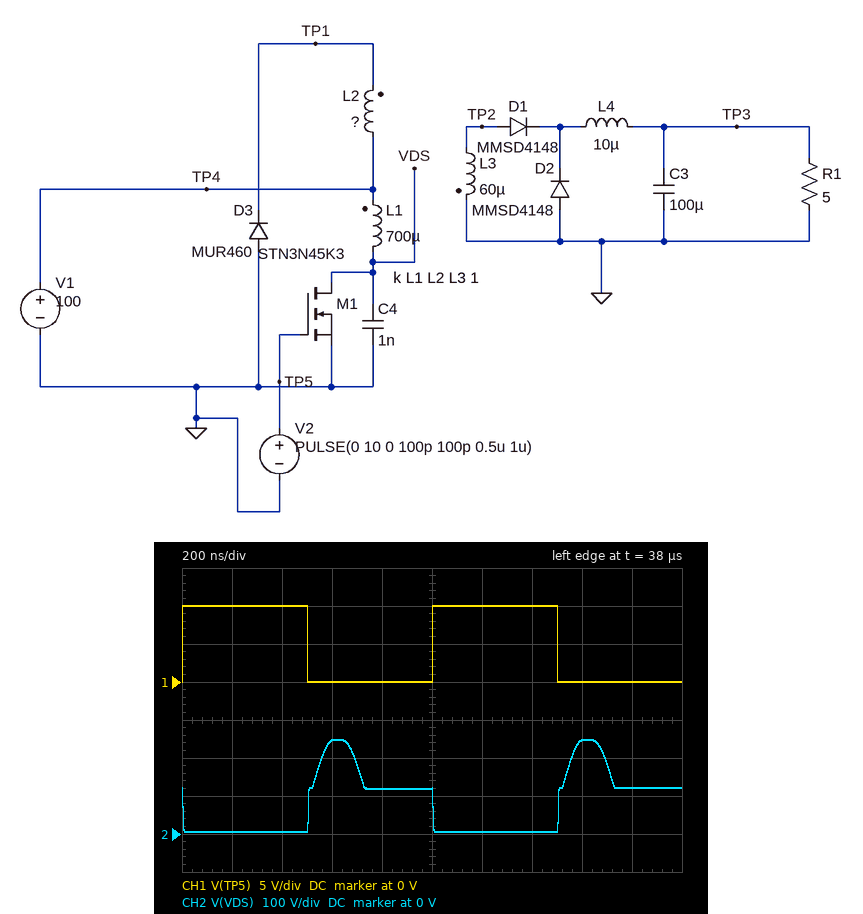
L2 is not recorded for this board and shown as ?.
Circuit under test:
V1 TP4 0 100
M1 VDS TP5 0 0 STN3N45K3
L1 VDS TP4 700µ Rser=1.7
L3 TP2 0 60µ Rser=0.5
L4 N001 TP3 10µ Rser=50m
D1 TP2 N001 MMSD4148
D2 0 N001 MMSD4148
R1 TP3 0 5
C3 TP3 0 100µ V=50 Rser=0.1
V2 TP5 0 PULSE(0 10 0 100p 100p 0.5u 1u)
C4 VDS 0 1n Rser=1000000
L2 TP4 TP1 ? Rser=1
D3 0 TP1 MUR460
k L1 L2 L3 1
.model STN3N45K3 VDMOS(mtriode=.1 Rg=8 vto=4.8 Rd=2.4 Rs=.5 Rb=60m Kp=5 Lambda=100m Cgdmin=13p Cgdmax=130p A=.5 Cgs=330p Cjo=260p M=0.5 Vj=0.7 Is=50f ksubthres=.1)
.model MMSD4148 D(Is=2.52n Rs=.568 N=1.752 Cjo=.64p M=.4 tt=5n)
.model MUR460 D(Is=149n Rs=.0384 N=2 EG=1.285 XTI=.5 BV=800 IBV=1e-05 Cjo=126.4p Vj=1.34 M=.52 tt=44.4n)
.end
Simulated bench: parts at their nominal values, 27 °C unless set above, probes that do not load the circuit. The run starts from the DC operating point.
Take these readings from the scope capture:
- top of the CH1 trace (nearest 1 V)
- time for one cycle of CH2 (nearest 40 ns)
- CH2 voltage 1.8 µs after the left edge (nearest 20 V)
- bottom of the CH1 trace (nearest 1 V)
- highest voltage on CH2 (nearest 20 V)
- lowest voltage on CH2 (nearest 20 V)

10 V
1.00 µs
120 V
0 V
240 V
0 V
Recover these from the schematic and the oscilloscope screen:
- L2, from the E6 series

330 µH
